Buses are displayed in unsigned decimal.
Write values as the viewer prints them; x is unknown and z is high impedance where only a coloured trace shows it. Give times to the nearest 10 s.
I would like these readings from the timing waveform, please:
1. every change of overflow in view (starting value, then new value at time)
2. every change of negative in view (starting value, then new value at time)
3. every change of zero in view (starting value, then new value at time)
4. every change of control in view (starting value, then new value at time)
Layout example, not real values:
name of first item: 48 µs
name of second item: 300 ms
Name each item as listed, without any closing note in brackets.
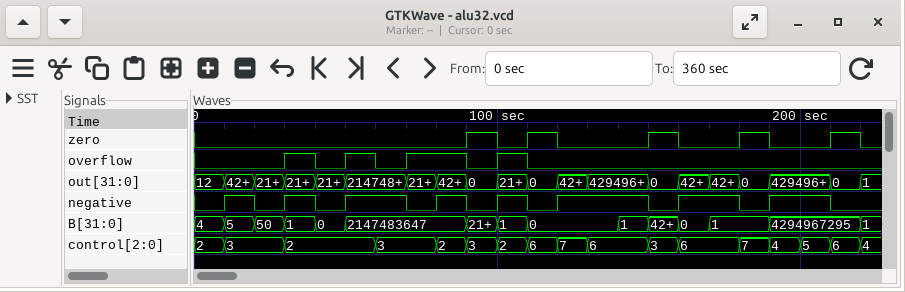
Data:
every change of overflow in view: 0, 1 at 30 s, 0 at 40 s, 1 at 50 s, 0 at 60 s, 1 at 70 s, 0 at 90 s, 1 at 100 s, 0 at 110 s
every change of negative in view: 0, 1 at 10 s, 0 at 20 s, 1 at 30 s, 0 at 40 s, 1 at 50 s, 0 at 70 s, 1 at 80 s, 0 at 90 s, 1 at 100 s, 0 at 110 s, 1 at 120 s, 0 at 150 s, 1 at 160 s, 0 at 180 s, 1 at 190 s, 0 at 210 s
every change of zero in view: 0, 1 at 90 s, 0 at 100 s, 1 at 110 s, 0 at 120 s, 1 at 150 s, 0 at 160 s, 1 at 180 s, 0 at 190 s, 1 at 210 s, 0 at 220 s
every change of control in view: 2, 3 at 10 s, 2 at 30 s, 3 at 60 s, 2 at 80 s, 3 at 90 s, 2 at 100 s, 6 at 110 s, 7 at 120 s, 6 at 130 s, 3 at 150 s, 6 at 160 s, 7 at 180 s, 4 at 190 s, 5 at 200 s, 6 at 210 s, 4 at 220 s
